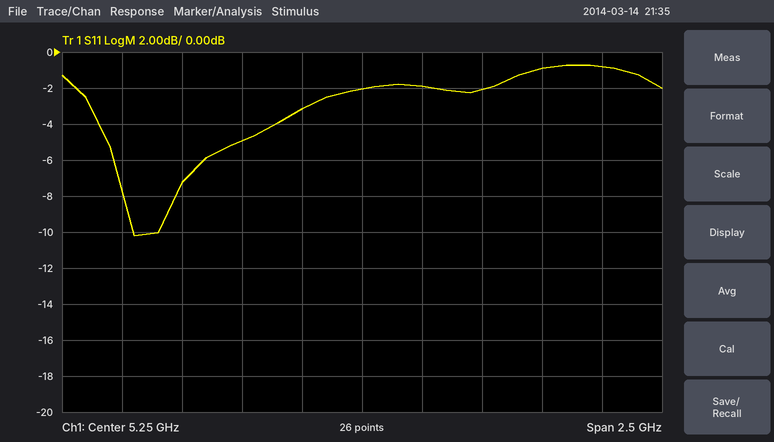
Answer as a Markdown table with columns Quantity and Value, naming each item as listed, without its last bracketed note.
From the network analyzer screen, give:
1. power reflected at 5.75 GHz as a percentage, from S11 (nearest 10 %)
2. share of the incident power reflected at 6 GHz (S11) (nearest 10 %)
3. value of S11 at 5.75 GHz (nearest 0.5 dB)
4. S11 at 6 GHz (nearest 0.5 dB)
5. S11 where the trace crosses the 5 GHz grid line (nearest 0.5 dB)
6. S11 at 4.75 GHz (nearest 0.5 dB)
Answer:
| Quantity | Value |
|---|---|
| power reflected at 5.75 GHz as a percentage, from S11 | 60 % |
| share of the incident power reflected at 6 GHz (S11) | 80 % |
| value of S11 at 5.75 GHz | -2.0 dB |
| S11 at 6 GHz | -1.0 dB |
| S11 where the trace crosses the 5 GHz grid line | -3.0 dB |
| S11 at 4.75 GHz | -5.0 dB |
